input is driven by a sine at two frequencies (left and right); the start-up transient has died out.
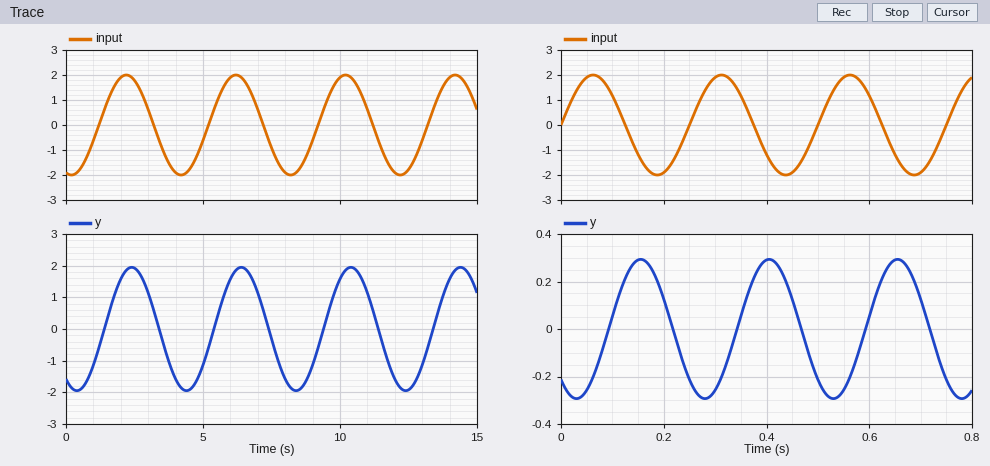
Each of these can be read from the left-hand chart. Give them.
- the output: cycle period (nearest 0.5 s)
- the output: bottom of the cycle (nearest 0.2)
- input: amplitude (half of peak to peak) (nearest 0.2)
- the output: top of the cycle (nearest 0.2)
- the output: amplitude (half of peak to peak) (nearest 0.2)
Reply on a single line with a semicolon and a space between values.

4.0 s; -2.0; 2.0; 2.0; 2.0
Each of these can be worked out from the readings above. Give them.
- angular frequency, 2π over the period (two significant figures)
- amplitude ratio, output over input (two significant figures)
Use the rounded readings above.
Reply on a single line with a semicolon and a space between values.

1.6 rad/s; 1.0
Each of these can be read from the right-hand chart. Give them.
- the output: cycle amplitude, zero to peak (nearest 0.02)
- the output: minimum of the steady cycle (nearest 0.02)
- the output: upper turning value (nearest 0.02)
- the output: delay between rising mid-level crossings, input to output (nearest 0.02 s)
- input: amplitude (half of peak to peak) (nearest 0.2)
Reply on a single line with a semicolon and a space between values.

0.30; -0.30; 0.30; 0.10 s; 2.0
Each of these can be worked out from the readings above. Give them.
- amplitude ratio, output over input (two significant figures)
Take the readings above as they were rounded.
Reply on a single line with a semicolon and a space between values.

0.15
